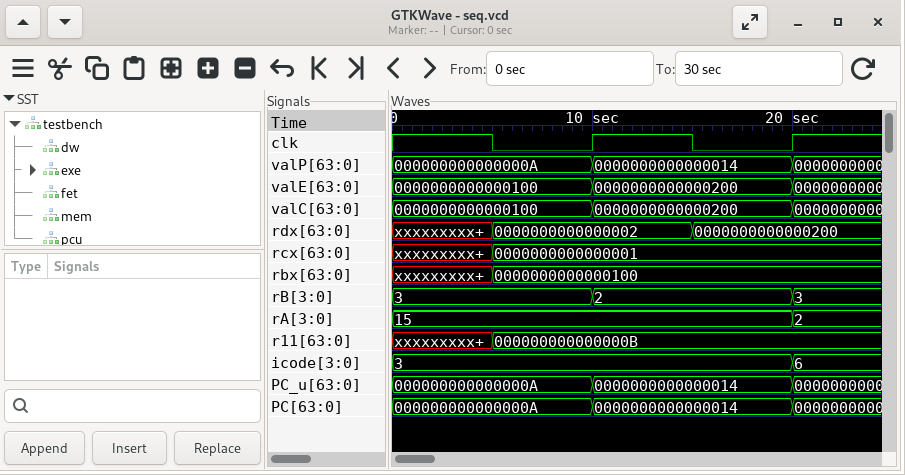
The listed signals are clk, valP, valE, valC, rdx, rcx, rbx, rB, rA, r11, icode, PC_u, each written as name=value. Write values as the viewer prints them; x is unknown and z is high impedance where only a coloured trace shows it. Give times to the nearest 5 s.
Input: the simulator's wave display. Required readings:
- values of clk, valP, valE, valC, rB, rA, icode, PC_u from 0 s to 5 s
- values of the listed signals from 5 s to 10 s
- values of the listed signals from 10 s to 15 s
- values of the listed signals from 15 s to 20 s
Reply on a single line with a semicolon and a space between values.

clk=1, valP=000000000000000A, valE=0000000000000100, valC=0000000000000100, rB=3, rA=15, icode=3, PC_u=000000000000000A; clk=0, valP=000000000000000A, valE=0000000000000100, valC=0000000000000100, rdx=0000000000000002, rcx=0000000000000001, rbx=0000000000000100, rB=3, rA=15, r11=000000000000000B, icode=3, PC_u=000000000000000A; clk=1, valP=0000000000000014, valE=0000000000000200, valC=0000000000000200, rdx=0000000000000002, rcx=0000000000000001, rbx=0000000000000100, rB=2, rA=15, r11=000000000000000B, icode=3, PC_u=0000000000000014; clk=0, valP=0000000000000014, valE=0000000000000200, valC=0000000000000200, rdx=0000000000000200, rcx=0000000000000001, rbx=0000000000000100, rB=2, rA=15, r11=000000000000000B, icode=3, PC_u=0000000000000014
